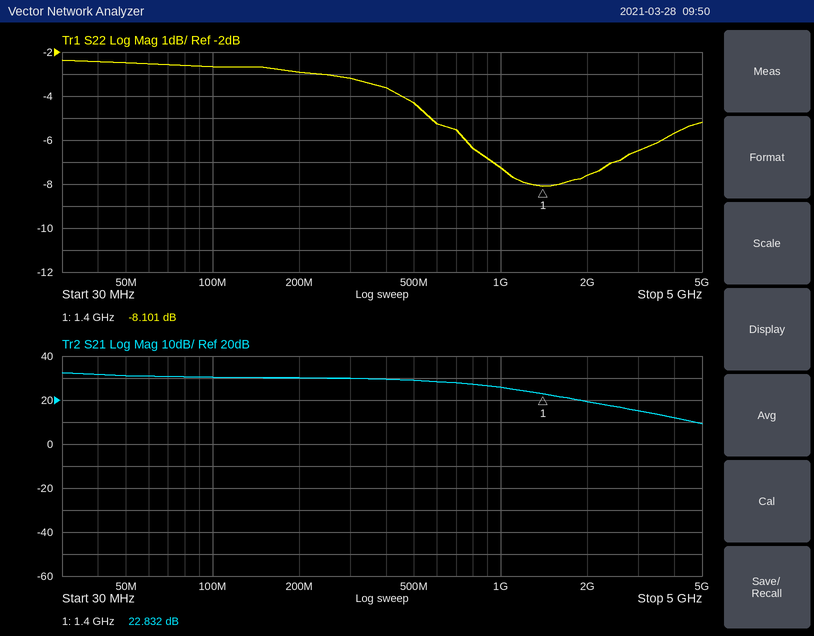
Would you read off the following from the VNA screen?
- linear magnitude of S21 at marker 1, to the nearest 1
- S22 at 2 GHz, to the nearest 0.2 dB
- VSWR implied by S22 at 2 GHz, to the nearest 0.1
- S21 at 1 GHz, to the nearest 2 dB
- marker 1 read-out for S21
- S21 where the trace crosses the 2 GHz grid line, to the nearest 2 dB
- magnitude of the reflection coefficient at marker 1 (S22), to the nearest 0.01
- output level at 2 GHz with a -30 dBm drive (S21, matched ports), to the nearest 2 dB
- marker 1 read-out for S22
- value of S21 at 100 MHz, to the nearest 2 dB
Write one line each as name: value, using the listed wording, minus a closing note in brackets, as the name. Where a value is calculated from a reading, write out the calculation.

linear magnitude of S21 at marker 1, to the nearest 1: 10^(22.832/20) ≈ 14
S22 at 2 GHz, to the nearest 0.2 dB: -7.6 dB
VSWR implied by S22 at 2 GHz, to the nearest 0.1: |Γ| = 10^(-7.6/20) = 0.4169; VSWR = (1 + 0.4169)/(1 − 0.4169) ≈ 2.4
S21 at 1 GHz, to the nearest 2 dB: 26 dB
marker 1 read-out for S21: 22.832 dB
S21 where the trace crosses the 2 GHz grid line, to the nearest 2 dB: 20 dB
magnitude of the reflection coefficient at marker 1 (S22), to the nearest 0.01: 10^(-8.101/20) ≈ 0.39
output level at 2 GHz with a -30 dBm drive (S21, matched ports), to the nearest 2 dB: -30 dBm + (20 dB) = -10 dBm
marker 1 read-out for S22: -8.101 dB
value of S21 at 100 MHz, to the nearest 2 dB: 30 dB
